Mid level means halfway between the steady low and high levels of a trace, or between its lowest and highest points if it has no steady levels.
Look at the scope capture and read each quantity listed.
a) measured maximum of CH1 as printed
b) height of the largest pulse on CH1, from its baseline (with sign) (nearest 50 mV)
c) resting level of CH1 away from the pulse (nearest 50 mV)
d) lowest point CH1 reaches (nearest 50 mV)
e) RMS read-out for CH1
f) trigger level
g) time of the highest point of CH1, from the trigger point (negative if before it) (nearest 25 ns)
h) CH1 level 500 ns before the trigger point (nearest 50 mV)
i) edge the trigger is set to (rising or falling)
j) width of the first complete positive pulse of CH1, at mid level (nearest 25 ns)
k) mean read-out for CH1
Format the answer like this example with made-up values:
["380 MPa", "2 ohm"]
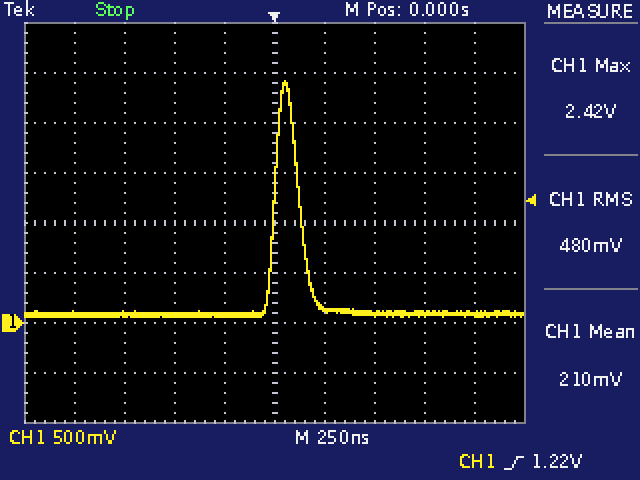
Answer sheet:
["2.42 V", "+2.35 V", "100 mV", "50 mV", "480 mV", "1.22 V", "+50 ns", "100 mV", "rising", "125 ns", "210 mV"]
